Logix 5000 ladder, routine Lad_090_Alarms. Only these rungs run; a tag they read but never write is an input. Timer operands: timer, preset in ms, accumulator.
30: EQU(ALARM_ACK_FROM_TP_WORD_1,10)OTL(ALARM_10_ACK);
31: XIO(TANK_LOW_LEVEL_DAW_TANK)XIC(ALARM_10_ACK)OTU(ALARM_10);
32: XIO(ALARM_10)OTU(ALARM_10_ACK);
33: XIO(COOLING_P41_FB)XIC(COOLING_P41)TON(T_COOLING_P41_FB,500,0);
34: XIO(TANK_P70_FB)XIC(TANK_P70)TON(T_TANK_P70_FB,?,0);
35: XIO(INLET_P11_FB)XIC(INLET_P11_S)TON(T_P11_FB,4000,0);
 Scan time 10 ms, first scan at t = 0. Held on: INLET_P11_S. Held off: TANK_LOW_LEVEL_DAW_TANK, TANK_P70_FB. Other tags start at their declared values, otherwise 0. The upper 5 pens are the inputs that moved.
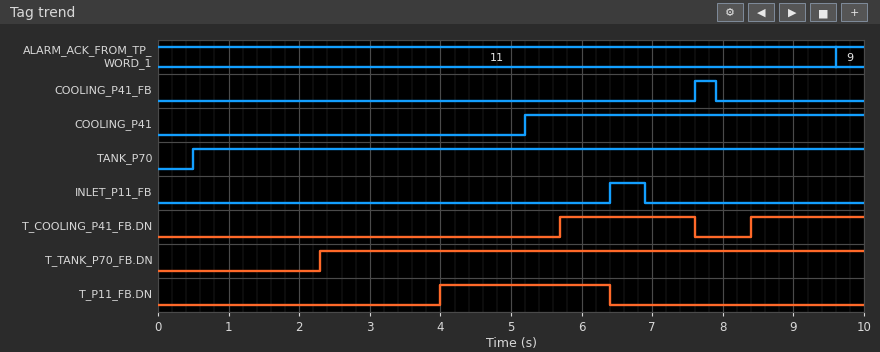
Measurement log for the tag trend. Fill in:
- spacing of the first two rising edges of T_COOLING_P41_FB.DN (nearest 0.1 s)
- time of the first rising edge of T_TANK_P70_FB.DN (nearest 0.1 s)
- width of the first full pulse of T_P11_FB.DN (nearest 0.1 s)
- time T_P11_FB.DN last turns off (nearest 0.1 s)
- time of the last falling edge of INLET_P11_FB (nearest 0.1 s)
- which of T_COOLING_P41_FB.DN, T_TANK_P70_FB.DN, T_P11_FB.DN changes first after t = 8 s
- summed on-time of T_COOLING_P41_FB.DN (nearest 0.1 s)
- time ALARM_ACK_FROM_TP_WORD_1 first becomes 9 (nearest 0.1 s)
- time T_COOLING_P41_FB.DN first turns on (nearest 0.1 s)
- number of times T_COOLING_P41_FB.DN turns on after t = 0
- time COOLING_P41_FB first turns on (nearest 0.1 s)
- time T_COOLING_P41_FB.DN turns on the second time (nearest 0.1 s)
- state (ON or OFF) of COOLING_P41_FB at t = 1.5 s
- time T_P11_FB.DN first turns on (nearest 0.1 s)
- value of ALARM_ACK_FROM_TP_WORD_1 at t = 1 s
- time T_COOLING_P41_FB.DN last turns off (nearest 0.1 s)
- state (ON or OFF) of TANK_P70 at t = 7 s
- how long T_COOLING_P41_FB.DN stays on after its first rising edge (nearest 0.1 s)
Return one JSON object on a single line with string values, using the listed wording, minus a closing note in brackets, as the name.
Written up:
{"spacing of the first two rising edges of T_COOLING_P41_FB.DN": "2.7 s", "time of the first rising edge of T_TANK_P70_FB.DN": "2.3 s", "width of the first full pulse of T_P11_FB.DN": "2.4 s", "time T_P11_FB.DN last turns off": "6.4 s", "time of the last falling edge of INLET_P11_FB": "6.9 s", "which of T_COOLING_P41_FB.DN, T_TANK_P70_FB.DN, T_P11_FB.DN changes first after t = 8 s": "T_COOLING_P41_FB.DN", "summed on-time of T_COOLING_P41_FB.DN": "3.5 s", "time ALARM_ACK_FROM_TP_WORD_1 first becomes 9": "9.6 s", "time T_COOLING_P41_FB.DN first turns on": "5.7 s", "number of times T_COOLING_P41_FB.DN turns on after t = 0": "2", "time COOLING_P41_FB first turns on": "7.6 s", "time T_COOLING_P41_FB.DN turns on the second time": "8.4 s", "state (ON or OFF) of COOLING_P41_FB at t = 1.5 s": "OFF", "time T_P11_FB.DN first turns on": "4.0 s", "value of ALARM_ACK_FROM_TP_WORD_1 at t = 1 s": "11", "time T_COOLING_P41_FB.DN last turns off": "7.6 s", "state (ON or OFF) of TANK_P70 at t = 7 s": "ON", "how long T_COOLING_P41_FB.DN stays on after its first rising edge": "1.9 s"}
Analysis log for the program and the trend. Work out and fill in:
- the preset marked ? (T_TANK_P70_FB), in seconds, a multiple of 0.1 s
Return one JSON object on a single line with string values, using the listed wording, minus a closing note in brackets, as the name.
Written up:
{"the preset marked ? (T_TANK_P70_FB), in seconds, a multiple of 0.1 s": "1.8 s"}
